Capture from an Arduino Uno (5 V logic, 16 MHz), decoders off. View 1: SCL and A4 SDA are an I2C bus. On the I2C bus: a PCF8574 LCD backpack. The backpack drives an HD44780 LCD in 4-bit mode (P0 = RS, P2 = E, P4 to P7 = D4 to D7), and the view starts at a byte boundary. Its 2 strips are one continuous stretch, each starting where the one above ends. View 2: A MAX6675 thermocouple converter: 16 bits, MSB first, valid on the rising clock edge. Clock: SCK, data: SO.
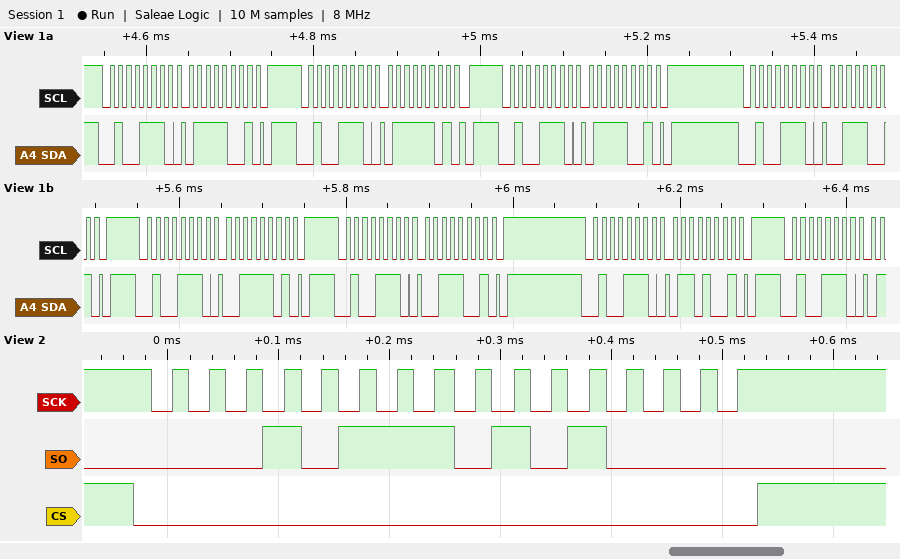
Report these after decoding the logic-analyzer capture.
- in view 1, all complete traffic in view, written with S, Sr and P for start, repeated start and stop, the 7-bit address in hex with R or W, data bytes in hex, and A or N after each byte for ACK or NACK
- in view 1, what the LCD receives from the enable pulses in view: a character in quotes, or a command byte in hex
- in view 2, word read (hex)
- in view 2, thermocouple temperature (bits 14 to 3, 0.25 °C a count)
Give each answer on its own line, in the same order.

S 27W A 79 A P S 27W A 7D A P S 27W A 79 A P S 27W A 39 A P S 27W A 3D A P S 27W A 39 A P S 27W A 69 A P S 27W A
's'
0x1750
186.50 °C
